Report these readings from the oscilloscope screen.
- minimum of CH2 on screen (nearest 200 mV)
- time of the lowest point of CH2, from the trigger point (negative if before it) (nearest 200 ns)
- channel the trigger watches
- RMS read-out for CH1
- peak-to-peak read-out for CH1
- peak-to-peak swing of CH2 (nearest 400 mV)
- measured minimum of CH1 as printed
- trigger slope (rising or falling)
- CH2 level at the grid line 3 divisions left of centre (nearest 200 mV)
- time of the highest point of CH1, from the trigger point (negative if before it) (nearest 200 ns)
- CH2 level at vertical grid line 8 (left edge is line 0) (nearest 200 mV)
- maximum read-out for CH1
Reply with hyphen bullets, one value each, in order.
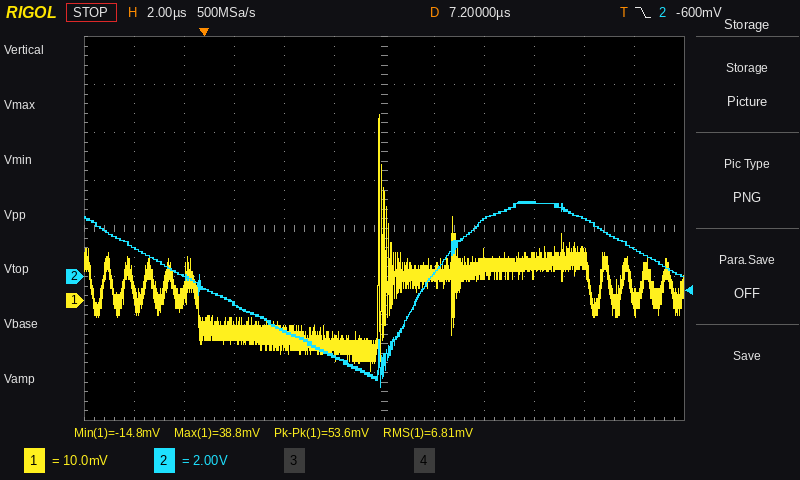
- -4.6 V
- +7.0 µs
- CH2
- 6.81 mV
- 53.6 mV
- 7.6 V
- -14.8 mV
- falling
- -1.2 V
- +7.0 µs
- 2.4 V
- 38.8 mV
